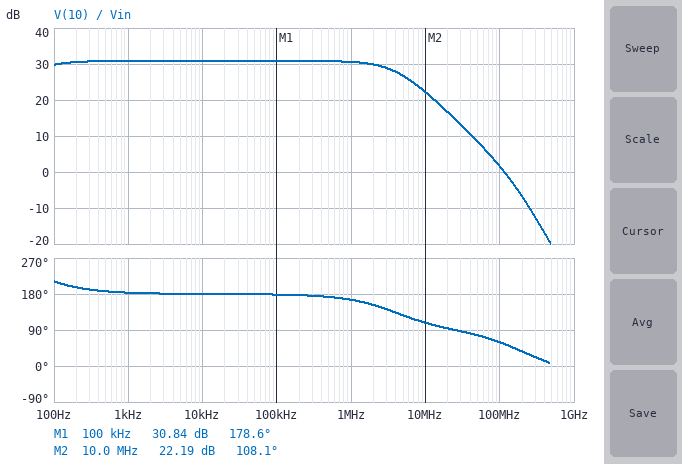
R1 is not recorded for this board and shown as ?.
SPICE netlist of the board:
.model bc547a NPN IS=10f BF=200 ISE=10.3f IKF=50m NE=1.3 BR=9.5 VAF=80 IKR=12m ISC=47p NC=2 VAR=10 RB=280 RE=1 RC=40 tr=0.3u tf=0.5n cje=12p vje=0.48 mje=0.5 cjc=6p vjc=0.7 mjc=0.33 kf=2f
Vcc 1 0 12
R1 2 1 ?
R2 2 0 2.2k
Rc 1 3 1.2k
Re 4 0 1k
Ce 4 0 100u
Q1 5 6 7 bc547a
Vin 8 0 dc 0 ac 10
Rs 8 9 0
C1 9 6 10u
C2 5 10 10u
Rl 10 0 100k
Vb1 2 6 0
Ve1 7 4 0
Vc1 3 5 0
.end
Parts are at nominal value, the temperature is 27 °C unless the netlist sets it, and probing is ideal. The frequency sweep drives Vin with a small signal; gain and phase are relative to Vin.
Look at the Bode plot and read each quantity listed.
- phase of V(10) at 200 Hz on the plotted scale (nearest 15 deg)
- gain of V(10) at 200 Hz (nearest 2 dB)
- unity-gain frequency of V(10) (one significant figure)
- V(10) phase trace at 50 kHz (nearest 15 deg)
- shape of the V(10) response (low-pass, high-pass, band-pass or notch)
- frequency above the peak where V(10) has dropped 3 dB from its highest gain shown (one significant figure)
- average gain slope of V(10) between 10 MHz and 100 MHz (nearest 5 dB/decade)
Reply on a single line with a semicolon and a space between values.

195 deg; 30 dB; 100 MHz; 180 deg; low-pass; 4 MHz; -20 dB/decade
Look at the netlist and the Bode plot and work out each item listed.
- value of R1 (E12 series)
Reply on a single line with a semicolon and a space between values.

15 kΩ
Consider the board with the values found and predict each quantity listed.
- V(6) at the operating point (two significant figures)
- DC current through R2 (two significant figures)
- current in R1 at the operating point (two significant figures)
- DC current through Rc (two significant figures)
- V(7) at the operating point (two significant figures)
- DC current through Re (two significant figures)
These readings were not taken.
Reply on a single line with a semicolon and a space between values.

1.5 V; 690 µA; 700 µA; 860 µA; 870 mV; 870 µA
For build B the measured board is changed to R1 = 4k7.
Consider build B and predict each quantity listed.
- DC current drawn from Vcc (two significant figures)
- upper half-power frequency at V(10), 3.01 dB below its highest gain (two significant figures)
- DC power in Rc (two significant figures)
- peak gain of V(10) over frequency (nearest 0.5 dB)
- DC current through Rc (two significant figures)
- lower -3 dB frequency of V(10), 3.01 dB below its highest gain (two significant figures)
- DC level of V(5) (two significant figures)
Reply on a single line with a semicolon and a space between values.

4.8 mA; 1.5 MHz; 11 mW; 39.5 dB; 3.1 mA; 140 Hz; 8.3 V
